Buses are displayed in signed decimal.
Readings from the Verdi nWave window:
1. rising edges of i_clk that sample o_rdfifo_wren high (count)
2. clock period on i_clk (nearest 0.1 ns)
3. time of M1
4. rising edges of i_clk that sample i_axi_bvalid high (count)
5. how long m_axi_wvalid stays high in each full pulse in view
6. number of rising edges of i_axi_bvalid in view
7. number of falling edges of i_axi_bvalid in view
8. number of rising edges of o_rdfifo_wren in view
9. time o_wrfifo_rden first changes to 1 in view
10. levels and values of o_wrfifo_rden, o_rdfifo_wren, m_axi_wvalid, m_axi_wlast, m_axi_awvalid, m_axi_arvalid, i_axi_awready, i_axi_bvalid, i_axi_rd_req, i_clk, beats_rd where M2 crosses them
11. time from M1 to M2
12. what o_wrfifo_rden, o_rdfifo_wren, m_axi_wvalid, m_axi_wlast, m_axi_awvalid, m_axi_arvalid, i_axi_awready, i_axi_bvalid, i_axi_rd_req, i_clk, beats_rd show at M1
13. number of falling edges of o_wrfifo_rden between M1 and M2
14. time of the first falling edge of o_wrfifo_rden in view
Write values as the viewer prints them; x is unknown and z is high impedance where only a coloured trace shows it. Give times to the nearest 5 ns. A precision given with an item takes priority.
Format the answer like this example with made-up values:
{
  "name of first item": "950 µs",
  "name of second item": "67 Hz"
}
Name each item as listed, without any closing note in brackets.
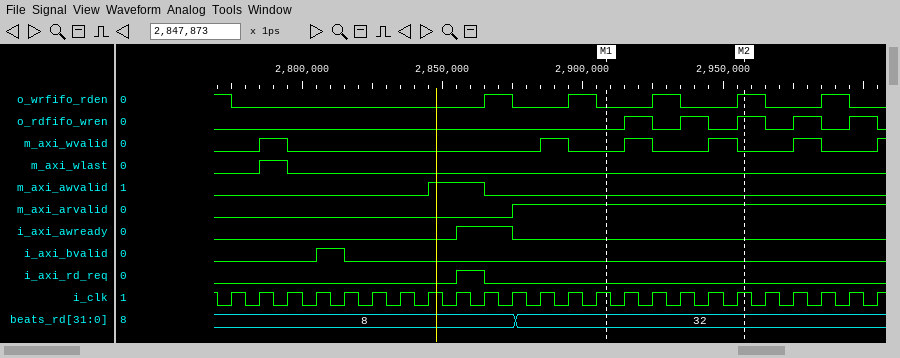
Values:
{
  "rising edges of i_clk that sample o_rdfifo_wren high": "5",
  "clock period on i_clk": "10 ns",
  "time of M1": "2910 ns",
  "rising edges of i_clk that sample i_axi_bvalid high": "1",
  "how long m_axi_wvalid stays high in each full pulse in view": "10 ns, 10 ns, 10 ns, 10 ns, 10 ns",
  "number of rising edges of i_axi_bvalid in view": "1",
  "number of falling edges of i_axi_bvalid in view": "1",
  "number of rising edges of o_rdfifo_wren in view": "5",
  "time o_wrfifo_rden first changes to 1 in view": "2865 ns",
  "levels and values of o_wrfifo_rden, o_rdfifo_wren, m_axi_wvalid, m_axi_wlast, m_axi_awvalid, m_axi_arvalid, i_axi_awready, i_axi_bvalid, i_axi_rd_req, i_clk, beats_rd where M2 crosses them": "o_wrfifo_rden=1, o_rdfifo_wren=1, m_axi_wvalid=0, m_axi_wlast=0, m_axi_awvalid=0, m_axi_arvalid=1, i_axi_awready=0, i_axi_bvalid=0, i_axi_rd_req=0, i_clk=1, beats_rd=32",
  "time from M1 to M2": "50 ns",
  "what o_wrfifo_rden, o_rdfifo_wren, m_axi_wvalid, m_axi_wlast, m_axi_awvalid, m_axi_arvalid, i_axi_awready, i_axi_bvalid, i_axi_rd_req, i_clk, beats_rd show at M1": "o_wrfifo_rden=0, o_rdfifo_wren=0, m_axi_wvalid=0, m_axi_wlast=0, m_axi_awvalid=0, m_axi_arvalid=1, i_axi_awready=0, i_axi_bvalid=0, i_axi_rd_req=0, i_clk=1, beats_rd=32",
  "number of falling edges of o_wrfifo_rden between M1 and M2": "1",
  "time of the first falling edge of o_wrfifo_rden in view": "2775 ns"
}
